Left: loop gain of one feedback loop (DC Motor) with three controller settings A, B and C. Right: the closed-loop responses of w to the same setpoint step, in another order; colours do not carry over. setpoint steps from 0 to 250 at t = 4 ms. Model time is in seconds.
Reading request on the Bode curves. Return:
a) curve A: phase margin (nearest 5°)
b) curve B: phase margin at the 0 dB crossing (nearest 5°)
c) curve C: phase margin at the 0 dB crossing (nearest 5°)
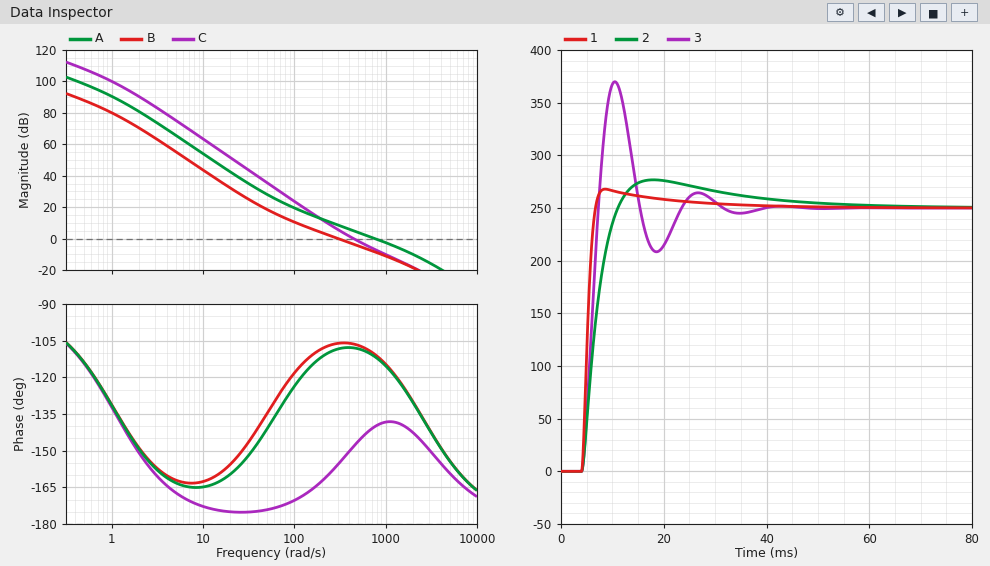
70°
75°
30°
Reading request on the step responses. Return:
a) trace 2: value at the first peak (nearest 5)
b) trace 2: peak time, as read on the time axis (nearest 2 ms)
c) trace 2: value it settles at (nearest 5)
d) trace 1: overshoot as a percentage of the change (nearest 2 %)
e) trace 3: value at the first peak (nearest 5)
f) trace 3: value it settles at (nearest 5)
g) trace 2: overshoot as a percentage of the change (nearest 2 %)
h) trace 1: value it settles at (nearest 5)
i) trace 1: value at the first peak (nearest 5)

275
18 ms
250
8 %
370
250
10 %
250
270
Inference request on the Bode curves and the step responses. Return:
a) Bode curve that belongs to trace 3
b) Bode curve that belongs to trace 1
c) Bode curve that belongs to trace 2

C
A
B
